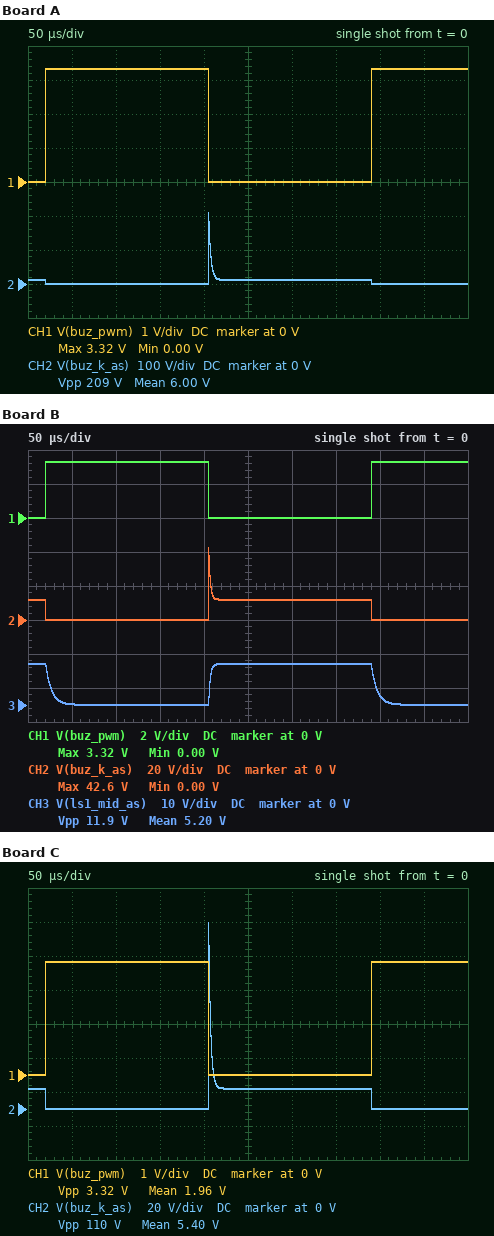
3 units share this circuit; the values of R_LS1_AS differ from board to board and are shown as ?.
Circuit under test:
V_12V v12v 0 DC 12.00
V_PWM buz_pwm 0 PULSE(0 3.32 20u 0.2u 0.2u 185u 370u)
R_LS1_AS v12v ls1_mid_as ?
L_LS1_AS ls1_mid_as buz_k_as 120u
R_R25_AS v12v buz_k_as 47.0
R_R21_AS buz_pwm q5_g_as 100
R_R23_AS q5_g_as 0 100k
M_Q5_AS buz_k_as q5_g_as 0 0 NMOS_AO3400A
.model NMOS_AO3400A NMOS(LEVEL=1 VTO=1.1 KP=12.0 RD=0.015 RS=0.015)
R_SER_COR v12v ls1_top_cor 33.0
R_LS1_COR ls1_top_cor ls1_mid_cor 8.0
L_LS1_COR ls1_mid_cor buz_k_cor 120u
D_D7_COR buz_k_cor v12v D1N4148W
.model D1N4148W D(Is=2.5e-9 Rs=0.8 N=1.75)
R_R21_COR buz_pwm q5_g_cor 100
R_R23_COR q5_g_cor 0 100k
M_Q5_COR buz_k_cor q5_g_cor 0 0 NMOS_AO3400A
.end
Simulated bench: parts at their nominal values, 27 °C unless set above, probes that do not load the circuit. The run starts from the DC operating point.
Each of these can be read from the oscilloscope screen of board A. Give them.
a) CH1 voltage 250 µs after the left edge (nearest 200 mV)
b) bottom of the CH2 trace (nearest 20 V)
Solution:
0 V
0 V
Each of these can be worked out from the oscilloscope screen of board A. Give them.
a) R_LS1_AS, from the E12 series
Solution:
2.7 Ω
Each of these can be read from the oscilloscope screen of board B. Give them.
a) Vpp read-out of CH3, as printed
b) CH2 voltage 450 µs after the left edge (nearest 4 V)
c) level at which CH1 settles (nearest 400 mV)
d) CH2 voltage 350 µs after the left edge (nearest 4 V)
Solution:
11.9 V
0 V
3.2 V
12 V
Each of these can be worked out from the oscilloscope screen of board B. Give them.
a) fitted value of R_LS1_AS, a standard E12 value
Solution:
18 Ω
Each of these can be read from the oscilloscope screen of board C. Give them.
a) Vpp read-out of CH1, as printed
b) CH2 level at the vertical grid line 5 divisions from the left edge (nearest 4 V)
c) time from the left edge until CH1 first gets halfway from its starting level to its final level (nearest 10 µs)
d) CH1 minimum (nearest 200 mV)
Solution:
3.32 V
12 V
20 µs
0 V
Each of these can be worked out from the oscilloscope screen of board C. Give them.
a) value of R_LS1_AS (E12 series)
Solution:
5.6 Ω
